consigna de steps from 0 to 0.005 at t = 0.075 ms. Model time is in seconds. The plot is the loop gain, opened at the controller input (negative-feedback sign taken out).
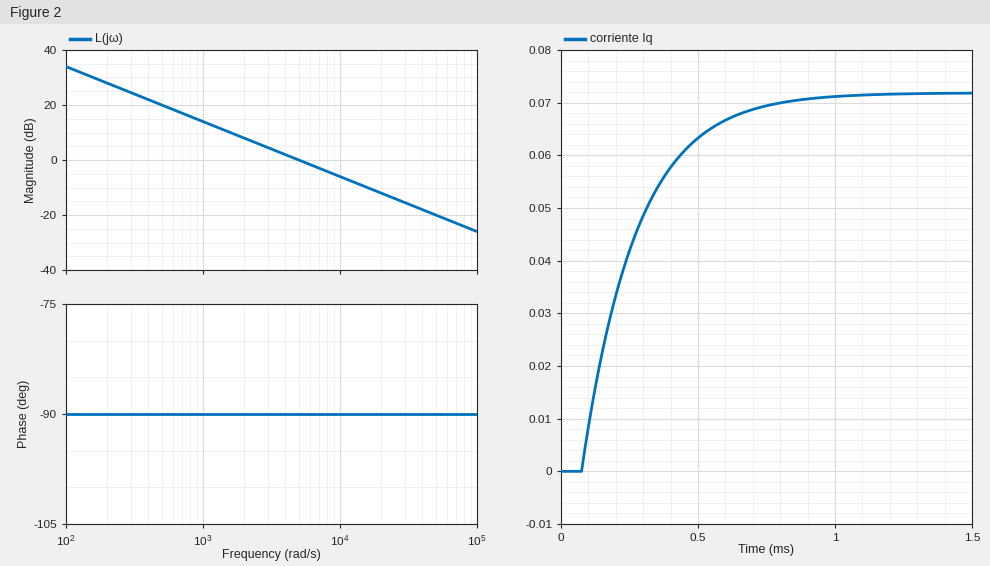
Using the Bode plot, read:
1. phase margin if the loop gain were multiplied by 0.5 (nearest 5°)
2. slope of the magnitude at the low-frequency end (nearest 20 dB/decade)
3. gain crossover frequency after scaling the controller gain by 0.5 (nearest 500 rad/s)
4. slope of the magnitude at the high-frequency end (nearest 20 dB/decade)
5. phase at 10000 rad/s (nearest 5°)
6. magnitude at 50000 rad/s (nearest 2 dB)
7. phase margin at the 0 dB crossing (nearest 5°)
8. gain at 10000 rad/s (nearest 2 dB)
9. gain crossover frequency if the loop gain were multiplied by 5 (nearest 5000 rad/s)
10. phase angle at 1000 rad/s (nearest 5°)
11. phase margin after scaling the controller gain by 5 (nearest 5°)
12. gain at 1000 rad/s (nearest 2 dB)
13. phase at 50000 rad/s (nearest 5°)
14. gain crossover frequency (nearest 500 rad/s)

90°
-20 dB/decade
2500 rad/s
-20 dB/decade
-90°
-20 dB
90°
-6 dB
25000 rad/s
-90°
90°
14 dB
-90°
5000 rad/s
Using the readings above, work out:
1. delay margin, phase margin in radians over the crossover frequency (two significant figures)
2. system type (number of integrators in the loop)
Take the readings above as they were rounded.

0.00031 s
1
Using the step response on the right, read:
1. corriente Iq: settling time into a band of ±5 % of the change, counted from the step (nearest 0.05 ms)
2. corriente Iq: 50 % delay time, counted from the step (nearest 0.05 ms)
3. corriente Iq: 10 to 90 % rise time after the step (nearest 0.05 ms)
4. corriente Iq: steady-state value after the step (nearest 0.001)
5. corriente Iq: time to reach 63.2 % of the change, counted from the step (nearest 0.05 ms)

0.60 ms
0.15 ms
0.45 ms
0.072
0.20 ms
